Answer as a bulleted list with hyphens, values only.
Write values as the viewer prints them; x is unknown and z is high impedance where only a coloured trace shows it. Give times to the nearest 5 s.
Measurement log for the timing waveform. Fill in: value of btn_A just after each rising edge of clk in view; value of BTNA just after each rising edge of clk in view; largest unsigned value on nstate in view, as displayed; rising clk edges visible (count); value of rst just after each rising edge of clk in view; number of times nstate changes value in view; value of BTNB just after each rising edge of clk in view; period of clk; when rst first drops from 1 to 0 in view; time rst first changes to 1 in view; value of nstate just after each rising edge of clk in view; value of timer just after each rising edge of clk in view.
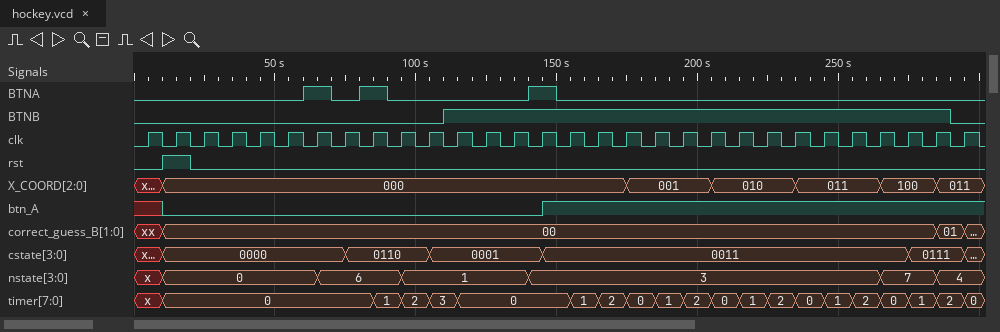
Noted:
- x 0 0 0 0 0 0 0 0 0 0 0 0 0 1 1 1 1 1 1 1 1 1 1 1 1 1 1 1 1
- 0 0 0 0 0 0 1 0 1 0 0 0 0 0 1 0 0 0 0 0 0 0 0 0 0 0 0 0 0 0
- 7
- 30
- 0 1 0 0 0 0 0 0 0 0 0 0 0 0 0 0 0 0 0 0 0 0 0 0 0 0 0 0 0 0
- 6
- 0 0 0 0 0 0 0 0 0 0 0 1 1 1 1 1 1 1 1 1 1 1 1 1 1 1 1 1 1 0
- 10 s
- 20 s
- 10 s
- x, 0, 0, 0, 0, 0, 6, 6, 6, 1, 1, 1, 1, 1, 3, 3, 3, 3, 3, 3, 3, 3, 3, 3, 3, 3, 7, 7, 4, 4
- x, 0, 0, 0, 0, 0, 0, 0, 1, 2, 3, 0, 0, 0, 0, 1, 2, 0, 1, 2, 0, 1, 2, 0, 1, 2, 0, 1, 2, 0
